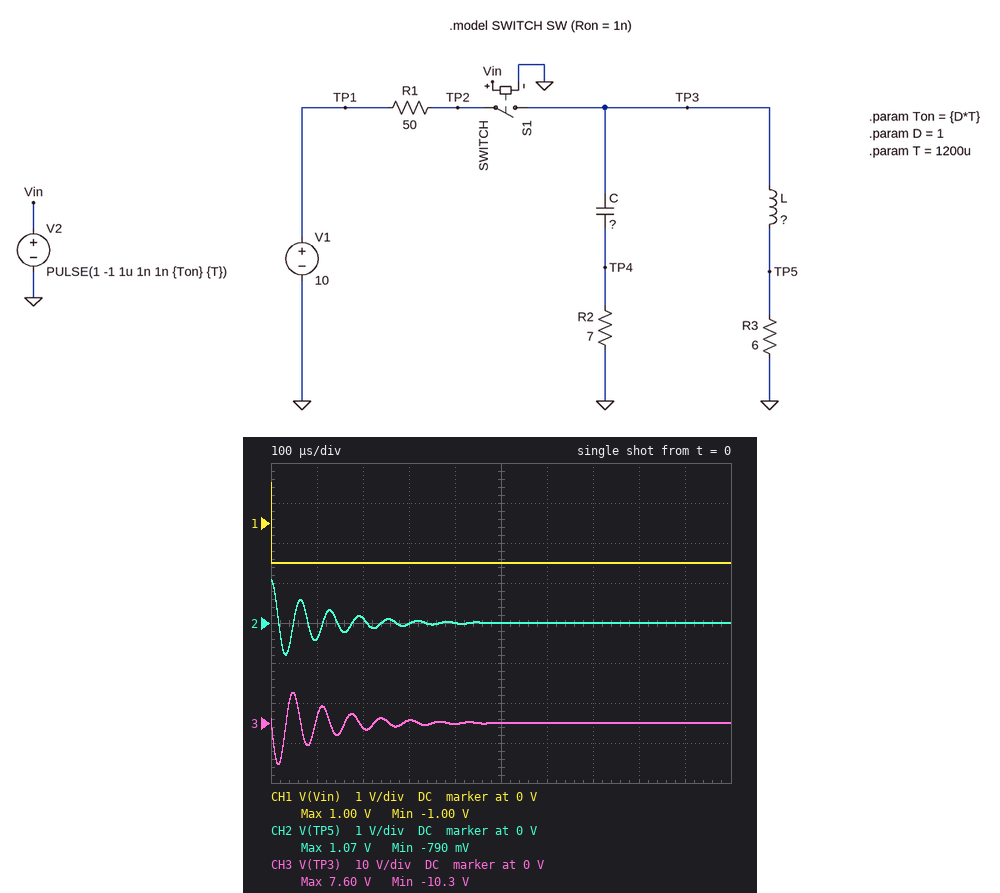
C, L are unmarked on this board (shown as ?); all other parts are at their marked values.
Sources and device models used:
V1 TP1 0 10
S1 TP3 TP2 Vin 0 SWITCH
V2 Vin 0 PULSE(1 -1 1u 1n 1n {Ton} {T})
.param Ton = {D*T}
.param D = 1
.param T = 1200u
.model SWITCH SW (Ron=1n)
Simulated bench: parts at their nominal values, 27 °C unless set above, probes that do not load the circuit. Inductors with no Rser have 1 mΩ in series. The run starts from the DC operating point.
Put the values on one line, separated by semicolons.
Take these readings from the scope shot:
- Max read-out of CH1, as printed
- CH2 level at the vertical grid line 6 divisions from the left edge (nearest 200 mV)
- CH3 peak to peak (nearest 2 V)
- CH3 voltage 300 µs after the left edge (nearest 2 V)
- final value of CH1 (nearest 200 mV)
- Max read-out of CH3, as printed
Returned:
1.00 V; 0 V; 18 V; 0 V; -1.0 V; 7.60 V
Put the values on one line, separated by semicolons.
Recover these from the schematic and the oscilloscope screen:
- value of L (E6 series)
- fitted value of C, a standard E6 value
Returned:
680 µH; 150 nF
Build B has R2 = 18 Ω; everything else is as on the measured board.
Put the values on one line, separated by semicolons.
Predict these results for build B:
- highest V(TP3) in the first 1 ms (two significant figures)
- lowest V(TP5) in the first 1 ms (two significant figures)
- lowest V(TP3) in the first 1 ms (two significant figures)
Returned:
5.3 V; -630 mV; -9.4 V
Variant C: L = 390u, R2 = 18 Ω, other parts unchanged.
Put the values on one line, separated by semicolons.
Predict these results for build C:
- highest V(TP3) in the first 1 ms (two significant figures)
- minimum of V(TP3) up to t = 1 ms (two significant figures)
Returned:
3.1 V; -6.7 V
